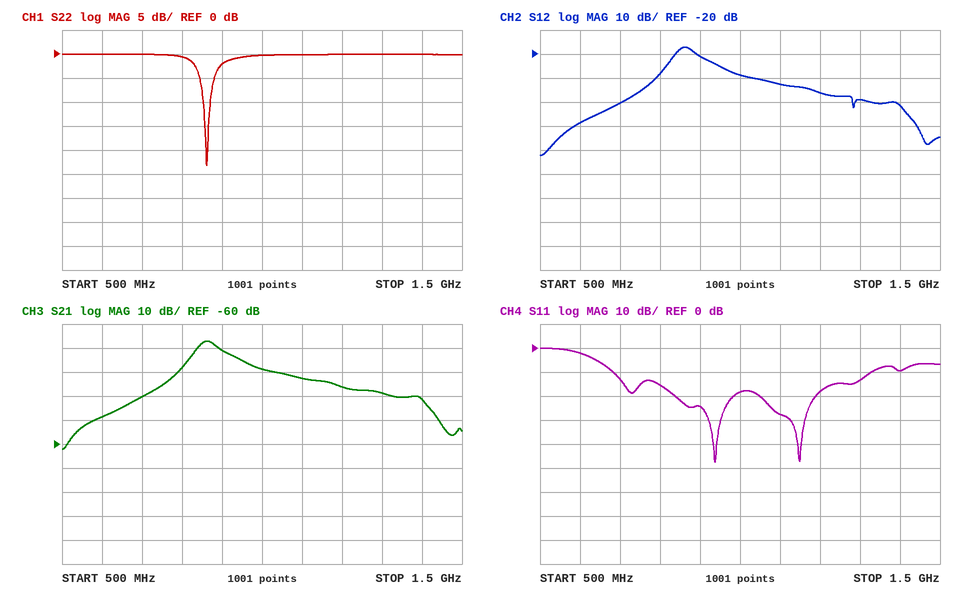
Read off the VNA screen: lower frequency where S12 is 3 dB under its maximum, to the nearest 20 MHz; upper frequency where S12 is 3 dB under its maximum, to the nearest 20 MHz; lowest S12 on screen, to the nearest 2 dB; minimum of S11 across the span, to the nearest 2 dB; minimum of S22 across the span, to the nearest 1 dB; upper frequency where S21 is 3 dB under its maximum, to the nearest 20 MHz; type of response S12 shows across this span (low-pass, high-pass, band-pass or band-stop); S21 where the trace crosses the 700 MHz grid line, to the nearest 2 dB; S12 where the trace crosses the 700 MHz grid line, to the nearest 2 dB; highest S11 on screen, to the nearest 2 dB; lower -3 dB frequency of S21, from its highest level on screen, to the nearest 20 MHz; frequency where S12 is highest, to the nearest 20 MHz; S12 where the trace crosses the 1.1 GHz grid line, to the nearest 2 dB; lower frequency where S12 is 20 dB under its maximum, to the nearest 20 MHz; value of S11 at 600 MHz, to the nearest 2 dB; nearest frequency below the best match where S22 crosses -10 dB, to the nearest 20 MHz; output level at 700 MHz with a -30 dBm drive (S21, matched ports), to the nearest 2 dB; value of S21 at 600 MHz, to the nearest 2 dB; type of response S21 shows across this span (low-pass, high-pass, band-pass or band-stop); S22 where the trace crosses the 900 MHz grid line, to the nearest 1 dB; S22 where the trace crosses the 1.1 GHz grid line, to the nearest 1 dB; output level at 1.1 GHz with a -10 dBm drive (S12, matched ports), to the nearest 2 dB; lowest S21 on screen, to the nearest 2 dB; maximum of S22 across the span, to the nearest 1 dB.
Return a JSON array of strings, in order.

["840 MHz", "900 MHz", "-62 dB", "-48 dB", "-23 dB", "900 MHz", "band-pass", "-40 dB", "-40 dB", "0 dB", "840 MHz", "860 MHz", "-32 dB", "740 MHz", "-2 dB", "860 MHz", "-70 dBm", "-48 dB", "band-pass", "-2 dB", "0 dB", "-42 dBm", "-62 dB", "0 dB"]
